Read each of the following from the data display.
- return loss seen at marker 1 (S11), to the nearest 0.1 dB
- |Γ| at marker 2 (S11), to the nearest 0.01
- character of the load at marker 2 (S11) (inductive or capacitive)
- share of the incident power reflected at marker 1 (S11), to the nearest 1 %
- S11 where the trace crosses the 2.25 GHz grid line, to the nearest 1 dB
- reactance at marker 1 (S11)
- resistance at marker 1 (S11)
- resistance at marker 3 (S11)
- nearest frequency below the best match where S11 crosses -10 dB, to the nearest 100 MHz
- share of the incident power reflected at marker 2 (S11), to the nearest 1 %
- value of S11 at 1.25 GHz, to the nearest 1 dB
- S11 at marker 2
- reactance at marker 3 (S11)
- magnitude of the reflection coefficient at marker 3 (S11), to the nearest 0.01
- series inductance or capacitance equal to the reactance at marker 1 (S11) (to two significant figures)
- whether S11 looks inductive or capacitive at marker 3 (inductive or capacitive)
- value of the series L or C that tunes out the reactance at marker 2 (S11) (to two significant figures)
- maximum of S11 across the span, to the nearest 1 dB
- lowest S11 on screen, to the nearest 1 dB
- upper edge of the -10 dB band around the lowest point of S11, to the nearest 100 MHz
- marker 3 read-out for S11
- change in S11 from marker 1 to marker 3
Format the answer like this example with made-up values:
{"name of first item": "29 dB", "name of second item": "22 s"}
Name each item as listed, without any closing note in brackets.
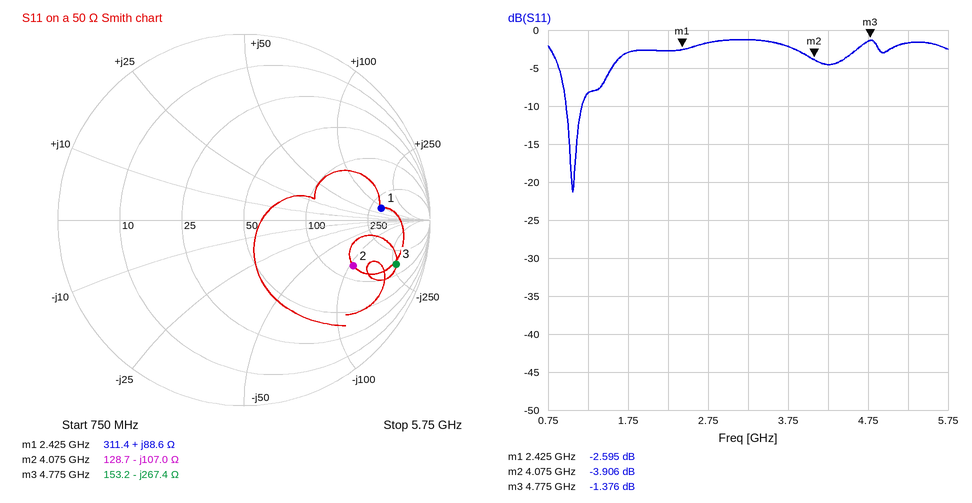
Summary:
{"return loss seen at marker 1 (S11), to the nearest 0.1 dB": "2.6 dB", "|Γ| at marker 2 (S11), to the nearest 0.01": "0.64", "character of the load at marker 2 (S11)": "capacitive", "share of the incident power reflected at marker 1 (S11), to the nearest 1 %": "55 %", "S11 where the trace crosses the 2.25 GHz grid line, to the nearest 1 dB": "-3 dB", "reactance at marker 1": "+88.6 Ω", "resistance at marker 1": "311.4 Ω", "resistance at marker 3": "153.2 Ω", "nearest frequency below the best match where S11 crosses -10 dB, to the nearest 100 MHz": "1.0 GHz", "share of the incident power reflected at marker 2 (S11), to the nearest 1 %": "41 %", "value of S11 at 1.25 GHz, to the nearest 1 dB": "-8 dB", "S11 at marker 2": "-3.906 dB", "reactance at marker 3": "-267.4 Ω", "magnitude of the reflection coefficient at marker 3 (S11), to the nearest 0.01": "0.85", "series inductance or capacitance equal to the reactance at marker 1 (S11)": "5.8 nH", "whether S11 looks inductive or capacitive at marker 3": "capacitive", "value of the series L or C that tunes out the reactance at marker 2 (S11)": "4.2 nH", "maximum of S11 across the span, to the nearest 1 dB": "-1 dB", "lowest S11 on screen, to the nearest 1 dB": "-21 dB", "upper edge of the -10 dB band around the lowest point of S11, to the nearest 100 MHz": "1.2 GHz", "marker 3 read-out for S11": "-1.376 dB", "change in S11 from marker 1 to marker 3": "1.219 dB"}
